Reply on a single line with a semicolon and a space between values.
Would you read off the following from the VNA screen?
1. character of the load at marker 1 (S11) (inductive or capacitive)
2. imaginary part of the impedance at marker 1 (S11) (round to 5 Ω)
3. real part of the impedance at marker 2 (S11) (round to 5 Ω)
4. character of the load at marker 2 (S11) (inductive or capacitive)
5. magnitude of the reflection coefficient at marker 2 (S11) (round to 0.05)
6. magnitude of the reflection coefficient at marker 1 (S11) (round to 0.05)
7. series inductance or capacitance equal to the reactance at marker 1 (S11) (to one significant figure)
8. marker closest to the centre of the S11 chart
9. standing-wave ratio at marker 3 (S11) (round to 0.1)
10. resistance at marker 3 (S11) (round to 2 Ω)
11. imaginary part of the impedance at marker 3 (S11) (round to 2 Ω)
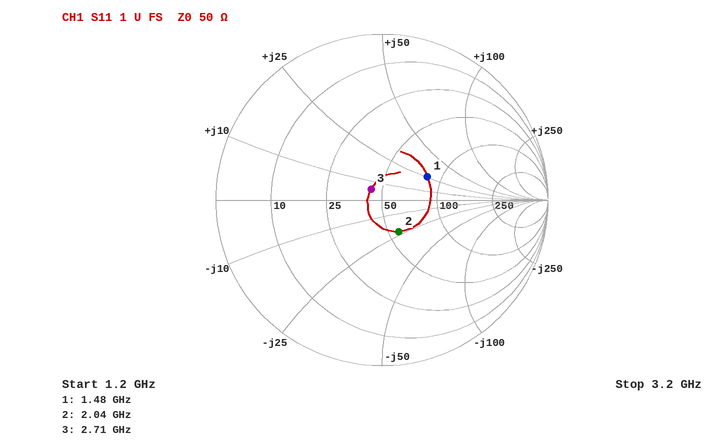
inductive; +25 Ω; 55 Ω; capacitive; 0.20; 0.30; 3 nH; marker 3; 1.2; 44 Ω; +6 Ω
